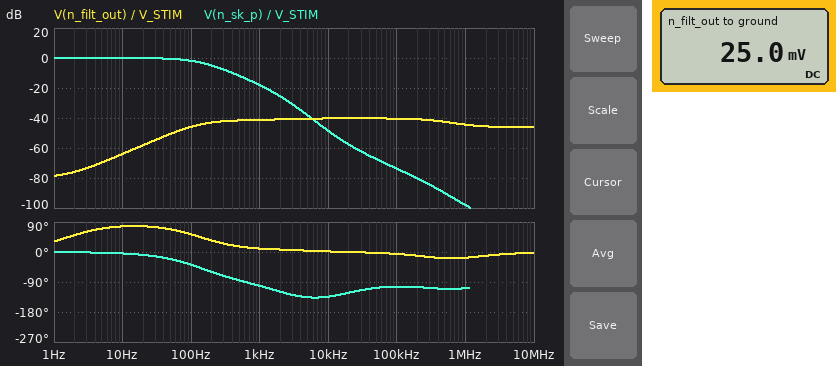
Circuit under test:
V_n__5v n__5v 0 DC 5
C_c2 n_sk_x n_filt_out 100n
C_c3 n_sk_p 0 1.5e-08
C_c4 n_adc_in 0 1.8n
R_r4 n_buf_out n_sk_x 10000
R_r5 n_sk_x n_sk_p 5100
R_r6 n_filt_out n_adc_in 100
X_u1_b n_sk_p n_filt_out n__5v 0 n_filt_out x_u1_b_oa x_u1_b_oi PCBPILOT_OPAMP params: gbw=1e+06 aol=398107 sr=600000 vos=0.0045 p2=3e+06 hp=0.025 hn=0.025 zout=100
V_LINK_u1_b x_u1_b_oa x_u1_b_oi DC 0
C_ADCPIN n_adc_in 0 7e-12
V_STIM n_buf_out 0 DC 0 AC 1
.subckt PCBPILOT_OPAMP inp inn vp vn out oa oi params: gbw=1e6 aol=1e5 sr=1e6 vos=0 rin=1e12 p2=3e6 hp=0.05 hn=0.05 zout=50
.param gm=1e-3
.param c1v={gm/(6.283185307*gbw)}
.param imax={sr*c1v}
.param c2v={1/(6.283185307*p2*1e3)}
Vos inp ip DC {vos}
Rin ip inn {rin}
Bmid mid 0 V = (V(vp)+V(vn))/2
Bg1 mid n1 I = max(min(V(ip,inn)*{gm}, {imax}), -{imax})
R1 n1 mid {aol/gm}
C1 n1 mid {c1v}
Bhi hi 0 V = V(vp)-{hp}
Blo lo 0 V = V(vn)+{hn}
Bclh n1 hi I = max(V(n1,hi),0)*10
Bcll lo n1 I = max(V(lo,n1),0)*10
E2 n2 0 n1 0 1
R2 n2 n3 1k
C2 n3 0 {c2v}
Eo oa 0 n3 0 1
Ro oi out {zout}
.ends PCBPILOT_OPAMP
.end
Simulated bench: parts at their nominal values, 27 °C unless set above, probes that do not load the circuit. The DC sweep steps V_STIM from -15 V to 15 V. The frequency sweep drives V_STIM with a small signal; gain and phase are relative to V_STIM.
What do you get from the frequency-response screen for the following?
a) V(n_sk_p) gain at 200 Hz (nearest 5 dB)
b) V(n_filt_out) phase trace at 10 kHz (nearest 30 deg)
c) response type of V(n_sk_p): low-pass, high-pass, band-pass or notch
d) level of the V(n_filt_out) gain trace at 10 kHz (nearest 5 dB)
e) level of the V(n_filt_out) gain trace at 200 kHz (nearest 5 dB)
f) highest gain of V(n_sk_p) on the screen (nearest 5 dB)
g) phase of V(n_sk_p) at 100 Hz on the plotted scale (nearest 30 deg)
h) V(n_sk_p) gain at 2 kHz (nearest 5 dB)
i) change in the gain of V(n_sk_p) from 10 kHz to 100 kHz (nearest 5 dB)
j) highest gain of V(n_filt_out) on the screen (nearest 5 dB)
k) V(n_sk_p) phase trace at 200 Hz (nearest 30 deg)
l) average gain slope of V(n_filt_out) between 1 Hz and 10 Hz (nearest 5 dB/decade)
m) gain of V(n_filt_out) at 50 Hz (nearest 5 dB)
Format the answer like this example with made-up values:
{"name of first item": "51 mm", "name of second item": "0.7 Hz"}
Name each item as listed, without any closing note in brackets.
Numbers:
{"V(n_sk_p) gain at 200 Hz": "-5 dB", "V(n_filt_out) phase trace at 10 kHz": "0 deg", "response type of V(n_sk_p): low-pass, high-pass, band-pass or notch": "low-pass", "level of the V(n_filt_out) gain trace at 10 kHz": "-40 dB", "level of the V(n_filt_out) gain trace at 200 kHz": "-40 dB", "highest gain of V(n_sk_p) on the screen": "0 dB", "phase of V(n_sk_p) at 100 Hz on the plotted scale": "-30 deg", "V(n_sk_p) gain at 2 kHz": "-25 dB", "change in the gain of V(n_sk_p) from 10 kHz to 100 kHz": "-25 dB", "highest gain of V(n_filt_out) on the screen": "-40 dB", "V(n_sk_p) phase trace at 200 Hz": "-60 deg", "average gain slope of V(n_filt_out) between 1 Hz and 10 Hz": "15 dB/decade", "gain of V(n_filt_out) at 50 Hz": "-50 dB"}
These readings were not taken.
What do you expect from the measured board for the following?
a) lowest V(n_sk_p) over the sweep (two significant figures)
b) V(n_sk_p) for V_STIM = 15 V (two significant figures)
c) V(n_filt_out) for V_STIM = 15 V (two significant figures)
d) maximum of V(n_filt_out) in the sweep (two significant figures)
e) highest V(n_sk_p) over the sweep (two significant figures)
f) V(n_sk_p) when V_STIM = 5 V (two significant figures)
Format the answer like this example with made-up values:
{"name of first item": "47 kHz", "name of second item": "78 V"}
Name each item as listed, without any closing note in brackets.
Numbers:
{"lowest V(n_sk_p) over the sweep": "-15 V", "V(n_sk_p) for V_STIM = 15 V": "15 V", "V(n_filt_out) for V_STIM = 15 V": "5.0 V", "maximum of V(n_filt_out) in the sweep": "5.0 V", "highest V(n_sk_p) over the sweep": "15 V", "V(n_sk_p) when V_STIM = 5 V": "5.0 V"}
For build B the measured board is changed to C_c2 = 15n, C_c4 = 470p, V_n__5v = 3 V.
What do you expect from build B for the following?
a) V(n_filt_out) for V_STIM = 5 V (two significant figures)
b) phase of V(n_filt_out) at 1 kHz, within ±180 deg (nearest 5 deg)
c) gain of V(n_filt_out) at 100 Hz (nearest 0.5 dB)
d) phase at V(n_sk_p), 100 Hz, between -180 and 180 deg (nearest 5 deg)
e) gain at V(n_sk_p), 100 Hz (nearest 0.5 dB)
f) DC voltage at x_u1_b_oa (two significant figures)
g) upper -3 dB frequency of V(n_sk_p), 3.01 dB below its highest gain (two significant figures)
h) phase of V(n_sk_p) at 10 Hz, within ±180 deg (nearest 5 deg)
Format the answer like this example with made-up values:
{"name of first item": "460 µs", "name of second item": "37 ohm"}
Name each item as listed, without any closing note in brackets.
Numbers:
{"V(n_filt_out) for V_STIM = 5 V": "3.0 V", "phase of V(n_filt_out) at 1 kHz, within ±180 deg": "40 deg", "gain of V(n_filt_out) at 100 Hz": "-60.5 dB", "phase at V(n_sk_p), 100 Hz, between -180 and 180 deg": "-15 deg", "gain at V(n_sk_p), 100 Hz": "0 dB", "DC voltage at x_u1_b_oa": "25 mV", "upper -3 dB frequency of V(n_sk_p), 3.01 dB below its highest gain": "460 Hz", "phase of V(n_sk_p) at 10 Hz, within ±180 deg": "0 deg"}
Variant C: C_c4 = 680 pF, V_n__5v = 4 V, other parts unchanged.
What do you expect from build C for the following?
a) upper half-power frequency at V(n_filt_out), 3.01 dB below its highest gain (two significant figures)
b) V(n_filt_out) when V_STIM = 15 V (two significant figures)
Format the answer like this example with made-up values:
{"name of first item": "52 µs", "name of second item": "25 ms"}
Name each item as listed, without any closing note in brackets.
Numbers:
{"upper half-power frequency at V(n_filt_out), 3.01 dB below its highest gain": "1.7 MHz", "V(n_filt_out) when V_STIM = 15 V": "4.0 V"}
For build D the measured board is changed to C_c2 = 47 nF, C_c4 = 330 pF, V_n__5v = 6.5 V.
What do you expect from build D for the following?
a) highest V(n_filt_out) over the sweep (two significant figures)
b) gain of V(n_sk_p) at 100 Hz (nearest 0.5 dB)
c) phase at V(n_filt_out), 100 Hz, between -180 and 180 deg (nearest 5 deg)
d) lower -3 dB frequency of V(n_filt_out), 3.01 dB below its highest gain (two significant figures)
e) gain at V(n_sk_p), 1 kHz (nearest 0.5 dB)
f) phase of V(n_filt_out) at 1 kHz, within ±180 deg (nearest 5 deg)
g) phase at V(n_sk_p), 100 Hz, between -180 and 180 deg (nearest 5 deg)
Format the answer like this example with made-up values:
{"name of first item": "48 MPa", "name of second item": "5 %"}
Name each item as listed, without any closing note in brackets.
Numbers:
{"highest V(n_filt_out) over the sweep": "6.5 V", "gain of V(n_sk_p) at 100 Hz": "-0.5 dB", "phase at V(n_filt_out), 100 Hz, between -180 and 180 deg": "65 deg", "lower -3 dB frequency of V(n_filt_out), 3.01 dB below its highest gain": "600 Hz", "gain at V(n_sk_p), 1 kHz": "-13.0 dB", "phase of V(n_filt_out) at 1 kHz, within ±180 deg": "20 deg", "phase at V(n_sk_p), 100 Hz, between -180 and 180 deg": "-25 deg"}
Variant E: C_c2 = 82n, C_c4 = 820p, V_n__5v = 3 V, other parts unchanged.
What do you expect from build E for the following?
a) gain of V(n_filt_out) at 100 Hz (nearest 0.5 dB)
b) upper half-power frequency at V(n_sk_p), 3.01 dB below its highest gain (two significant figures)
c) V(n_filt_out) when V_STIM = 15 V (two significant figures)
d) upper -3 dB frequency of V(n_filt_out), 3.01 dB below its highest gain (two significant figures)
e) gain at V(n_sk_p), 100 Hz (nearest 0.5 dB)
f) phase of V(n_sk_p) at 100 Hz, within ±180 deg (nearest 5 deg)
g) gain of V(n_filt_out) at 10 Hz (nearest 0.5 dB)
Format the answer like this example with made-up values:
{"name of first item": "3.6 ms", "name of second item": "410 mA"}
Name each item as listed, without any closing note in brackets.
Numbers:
{"gain of V(n_filt_out) at 100 Hz": "-47.0 dB", "upper half-power frequency at V(n_sk_p), 3.01 dB below its highest gain": "160 Hz", "V(n_filt_out) when V_STIM = 15 V": "3.0 V", "upper -3 dB frequency of V(n_filt_out), 3.01 dB below its highest gain": "1.4 MHz", "gain at V(n_sk_p), 100 Hz": "-1.5 dB", "phase of V(n_sk_p) at 100 Hz, within ±180 deg": "-35 deg", "gain of V(n_filt_out) at 10 Hz": "-65.5 dB"}
